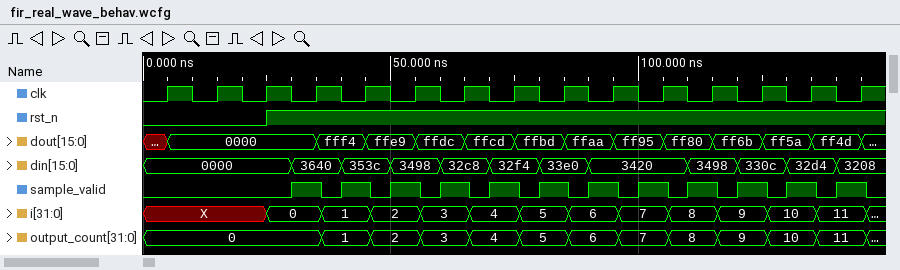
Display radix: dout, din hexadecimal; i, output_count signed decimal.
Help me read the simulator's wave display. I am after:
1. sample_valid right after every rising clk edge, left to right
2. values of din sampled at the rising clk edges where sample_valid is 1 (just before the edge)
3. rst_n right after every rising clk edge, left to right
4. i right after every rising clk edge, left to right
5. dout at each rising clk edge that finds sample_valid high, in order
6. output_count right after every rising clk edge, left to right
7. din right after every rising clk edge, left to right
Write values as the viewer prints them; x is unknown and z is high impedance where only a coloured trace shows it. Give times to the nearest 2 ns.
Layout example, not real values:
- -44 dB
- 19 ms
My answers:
- 0 0 0 1 1 1 1 1 1 1 1 1 1 1 1
- 3640, 353c, 3498, 32c8, 32f4, 33e0, 3420, 3420, 3498, 330c, 32d4, 3208
- 0 0 1 1 1 1 1 1 1 1 1 1 1 1 1
- X, X, 0, 0, 1, 2, 3, 4, 5, 6, 7, 8, 9, 10, 11
- 0000, fff4, ffe9, ffdc, ffcd, ffbd, ffaa, ff95, ff80, ff6b, ff5a, ff4d
- 0, 0, 0, 0, 1, 2, 3, 4, 5, 6, 7, 8, 9, 10, 11
- 0000, 0000, 0000, 3640, 353c, 3498, 32c8, 32f4, 33e0, 3420, 3420, 3498, 330c, 32d4, 3208
